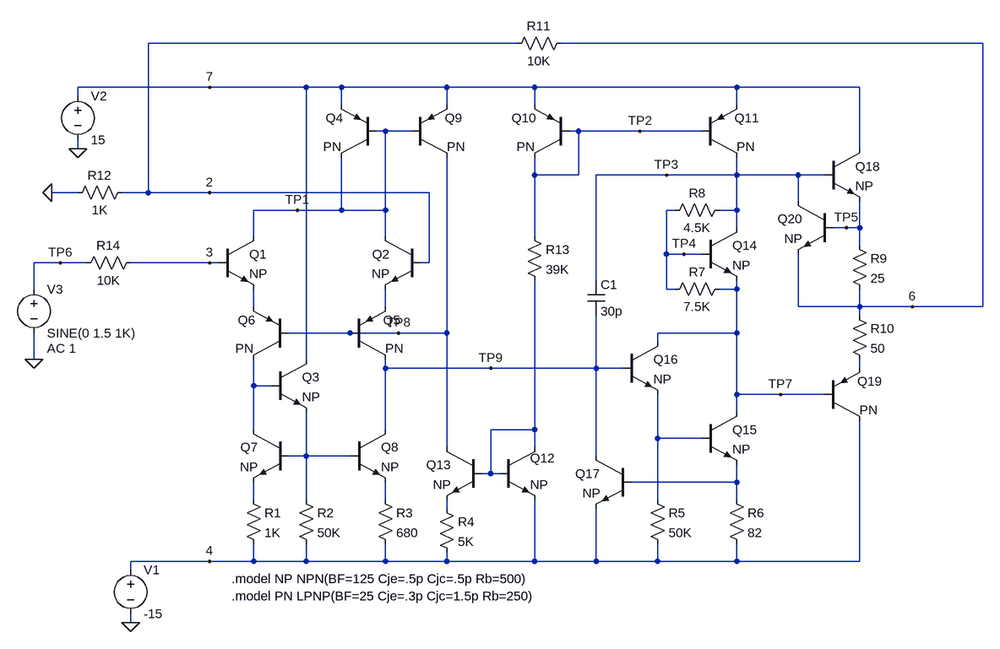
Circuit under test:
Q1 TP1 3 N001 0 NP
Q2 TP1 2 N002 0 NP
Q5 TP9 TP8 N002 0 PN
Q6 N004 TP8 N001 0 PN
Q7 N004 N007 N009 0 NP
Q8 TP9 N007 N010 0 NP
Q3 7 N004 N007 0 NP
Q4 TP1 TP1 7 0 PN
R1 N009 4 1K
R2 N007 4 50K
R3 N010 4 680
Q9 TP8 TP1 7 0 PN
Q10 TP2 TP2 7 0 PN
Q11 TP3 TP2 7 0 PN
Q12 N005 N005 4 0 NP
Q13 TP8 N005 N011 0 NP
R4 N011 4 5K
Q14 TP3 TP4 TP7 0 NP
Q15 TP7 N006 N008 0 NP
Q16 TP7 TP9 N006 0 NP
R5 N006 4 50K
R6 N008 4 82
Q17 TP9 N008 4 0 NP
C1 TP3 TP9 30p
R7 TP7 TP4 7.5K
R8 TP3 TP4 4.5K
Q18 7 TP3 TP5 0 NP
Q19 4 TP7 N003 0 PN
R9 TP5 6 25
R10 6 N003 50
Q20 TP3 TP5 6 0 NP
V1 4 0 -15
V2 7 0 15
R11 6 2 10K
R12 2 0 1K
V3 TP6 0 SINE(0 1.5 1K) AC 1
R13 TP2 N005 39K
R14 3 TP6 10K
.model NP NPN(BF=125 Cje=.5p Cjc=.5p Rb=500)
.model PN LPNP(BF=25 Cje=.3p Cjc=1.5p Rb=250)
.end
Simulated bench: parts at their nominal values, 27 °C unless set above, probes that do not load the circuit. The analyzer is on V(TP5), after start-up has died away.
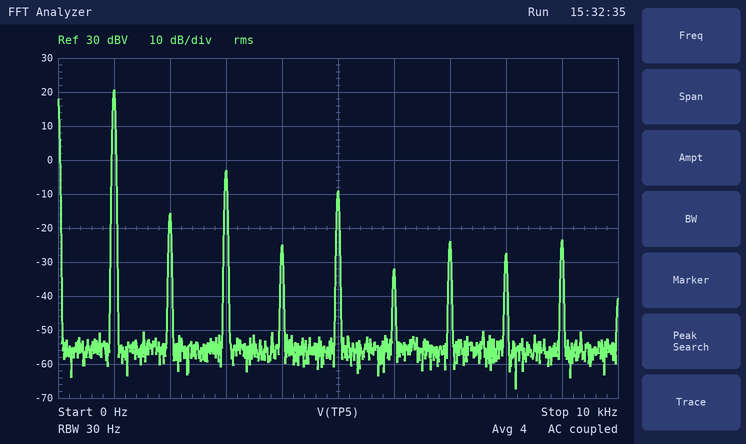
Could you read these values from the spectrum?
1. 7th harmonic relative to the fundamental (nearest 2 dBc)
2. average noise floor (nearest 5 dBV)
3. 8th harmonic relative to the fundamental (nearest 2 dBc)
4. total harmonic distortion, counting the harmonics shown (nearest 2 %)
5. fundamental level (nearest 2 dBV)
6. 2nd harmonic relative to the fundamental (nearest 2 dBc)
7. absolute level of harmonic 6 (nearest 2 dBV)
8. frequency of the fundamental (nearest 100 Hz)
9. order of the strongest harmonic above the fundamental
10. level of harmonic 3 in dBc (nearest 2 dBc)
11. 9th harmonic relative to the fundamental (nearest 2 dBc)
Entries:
-44 dBc
-55 dBV
-48 dBc
8 %
20 dBV
-36 dBc
-32 dBV
1.0 kHz
3
-24 dBc
-44 dBc
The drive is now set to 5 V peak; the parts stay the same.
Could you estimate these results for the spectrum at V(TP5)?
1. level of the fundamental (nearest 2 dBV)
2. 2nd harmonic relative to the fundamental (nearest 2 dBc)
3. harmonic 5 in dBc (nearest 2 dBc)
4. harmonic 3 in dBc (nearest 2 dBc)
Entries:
22 dBV
-44 dBc
-16 dBc
-10 dBc
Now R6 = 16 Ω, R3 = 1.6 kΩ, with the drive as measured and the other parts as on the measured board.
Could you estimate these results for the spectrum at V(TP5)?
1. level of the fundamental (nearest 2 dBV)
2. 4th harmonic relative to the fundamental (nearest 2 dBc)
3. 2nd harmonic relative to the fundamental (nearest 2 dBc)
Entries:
20 dBV
-44 dBc
-34 dBc
